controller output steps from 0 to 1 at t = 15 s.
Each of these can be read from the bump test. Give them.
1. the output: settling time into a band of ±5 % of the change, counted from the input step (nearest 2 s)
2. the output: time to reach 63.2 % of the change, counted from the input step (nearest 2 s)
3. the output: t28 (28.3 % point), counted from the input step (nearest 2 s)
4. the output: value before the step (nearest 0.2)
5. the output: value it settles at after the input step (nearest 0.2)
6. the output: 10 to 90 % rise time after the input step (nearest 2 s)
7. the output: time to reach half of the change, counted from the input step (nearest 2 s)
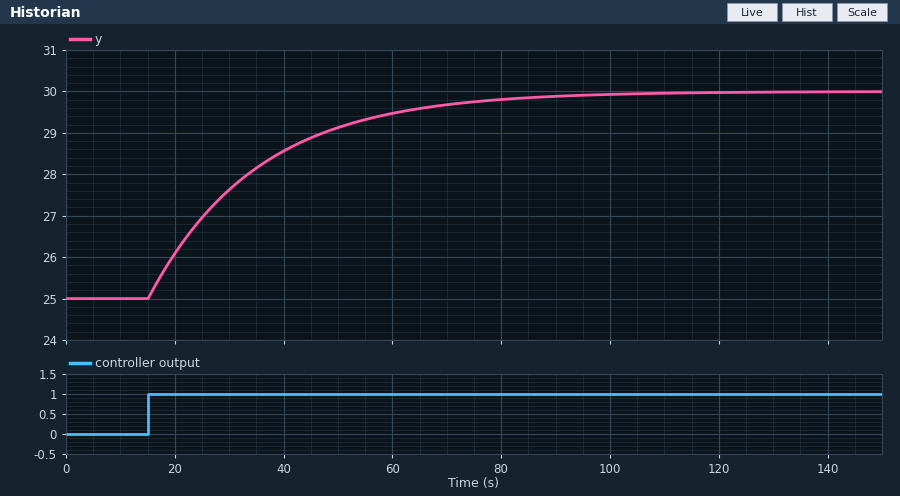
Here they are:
60 s
20 s
6 s
25.0
30.0
44 s
14 s
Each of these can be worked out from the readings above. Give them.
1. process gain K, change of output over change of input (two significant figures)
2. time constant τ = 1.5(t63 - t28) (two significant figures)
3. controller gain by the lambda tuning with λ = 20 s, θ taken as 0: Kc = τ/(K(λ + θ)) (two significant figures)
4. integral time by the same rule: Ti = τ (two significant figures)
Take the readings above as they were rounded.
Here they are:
5.0
21 s
0.21
21 s
